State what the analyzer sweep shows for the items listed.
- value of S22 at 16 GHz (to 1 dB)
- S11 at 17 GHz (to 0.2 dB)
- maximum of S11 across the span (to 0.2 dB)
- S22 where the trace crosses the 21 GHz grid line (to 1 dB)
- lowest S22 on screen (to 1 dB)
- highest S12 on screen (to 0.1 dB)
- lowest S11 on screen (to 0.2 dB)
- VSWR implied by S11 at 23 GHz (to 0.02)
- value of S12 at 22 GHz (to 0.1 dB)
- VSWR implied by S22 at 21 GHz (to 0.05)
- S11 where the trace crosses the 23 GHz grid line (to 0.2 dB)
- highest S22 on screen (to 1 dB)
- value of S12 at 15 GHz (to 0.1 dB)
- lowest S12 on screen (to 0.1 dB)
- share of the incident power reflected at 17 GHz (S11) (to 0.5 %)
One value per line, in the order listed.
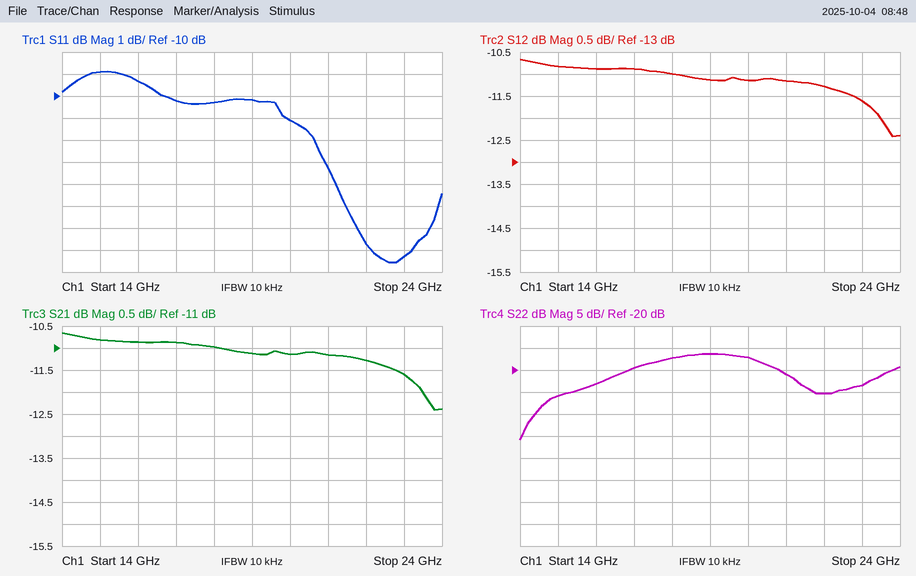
-23 dB
-10.2 dB
-8.8 dB
-21 dB
-36 dB
-10.7 dB
-17.6 dB
1.32
-11.3 dB
1.20
-17.2 dB
-16 dB
-10.8 dB
-12.4 dB
9.5 %
